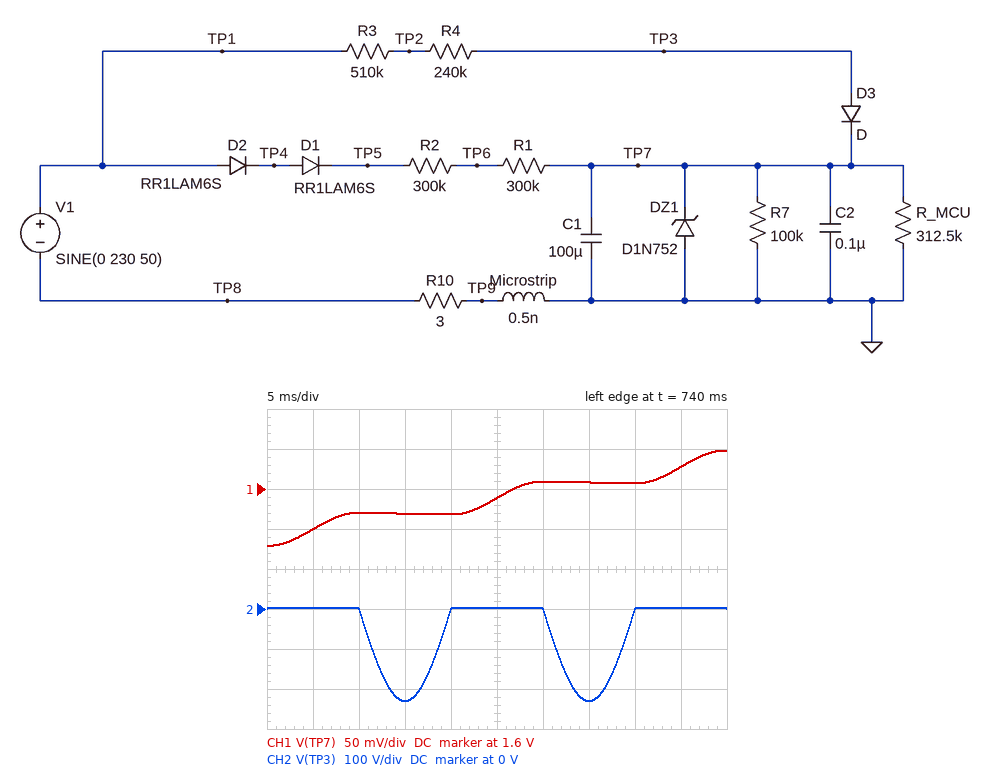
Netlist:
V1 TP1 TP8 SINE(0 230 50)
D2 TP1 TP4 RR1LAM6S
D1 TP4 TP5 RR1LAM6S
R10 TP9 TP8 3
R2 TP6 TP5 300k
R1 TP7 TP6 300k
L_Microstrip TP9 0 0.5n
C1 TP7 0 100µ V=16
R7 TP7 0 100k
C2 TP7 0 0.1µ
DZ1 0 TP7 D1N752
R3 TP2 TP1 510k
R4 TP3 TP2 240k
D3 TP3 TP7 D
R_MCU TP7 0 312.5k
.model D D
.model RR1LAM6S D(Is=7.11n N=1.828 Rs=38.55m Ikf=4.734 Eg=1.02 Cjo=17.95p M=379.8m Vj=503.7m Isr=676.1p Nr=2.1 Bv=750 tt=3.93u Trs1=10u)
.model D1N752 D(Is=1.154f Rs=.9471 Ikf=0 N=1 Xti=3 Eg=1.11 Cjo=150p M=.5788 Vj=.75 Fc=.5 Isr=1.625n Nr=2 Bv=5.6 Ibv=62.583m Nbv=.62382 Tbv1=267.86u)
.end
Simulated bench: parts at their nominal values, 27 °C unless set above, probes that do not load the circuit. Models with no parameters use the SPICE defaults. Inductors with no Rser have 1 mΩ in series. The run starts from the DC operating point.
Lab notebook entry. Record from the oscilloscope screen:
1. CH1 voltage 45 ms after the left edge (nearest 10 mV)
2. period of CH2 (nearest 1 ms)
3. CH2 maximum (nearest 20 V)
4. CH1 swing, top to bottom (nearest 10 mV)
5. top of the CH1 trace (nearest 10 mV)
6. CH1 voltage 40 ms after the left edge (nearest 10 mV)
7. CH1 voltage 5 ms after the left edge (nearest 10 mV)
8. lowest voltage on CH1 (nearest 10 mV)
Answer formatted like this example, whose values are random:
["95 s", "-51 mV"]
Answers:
["1.63 V", "20 ms", "0 V", "120 mV", "1.65 V", "1.61 V", "1.55 V", "1.53 V"]
